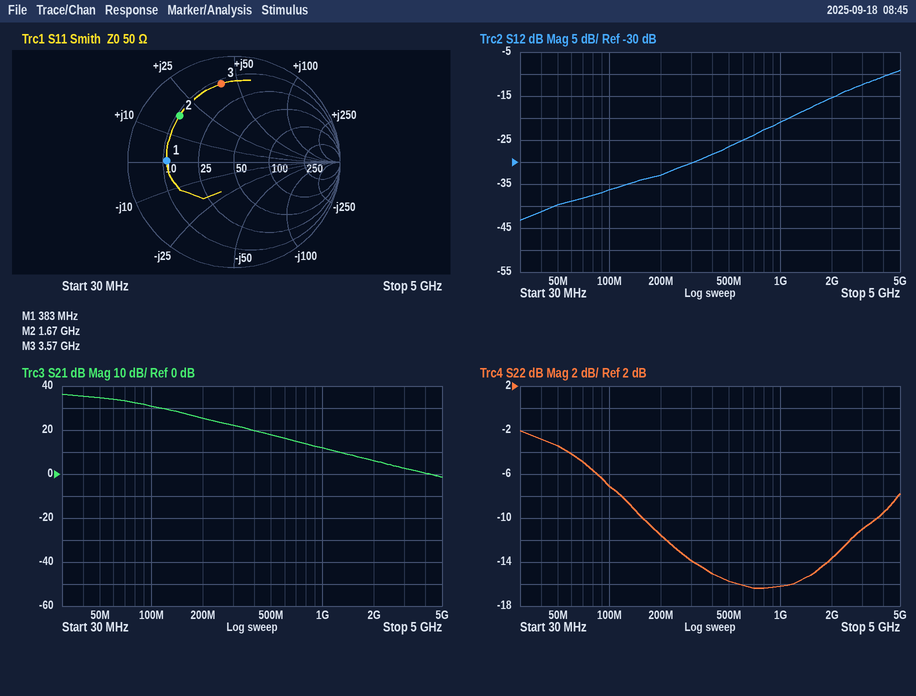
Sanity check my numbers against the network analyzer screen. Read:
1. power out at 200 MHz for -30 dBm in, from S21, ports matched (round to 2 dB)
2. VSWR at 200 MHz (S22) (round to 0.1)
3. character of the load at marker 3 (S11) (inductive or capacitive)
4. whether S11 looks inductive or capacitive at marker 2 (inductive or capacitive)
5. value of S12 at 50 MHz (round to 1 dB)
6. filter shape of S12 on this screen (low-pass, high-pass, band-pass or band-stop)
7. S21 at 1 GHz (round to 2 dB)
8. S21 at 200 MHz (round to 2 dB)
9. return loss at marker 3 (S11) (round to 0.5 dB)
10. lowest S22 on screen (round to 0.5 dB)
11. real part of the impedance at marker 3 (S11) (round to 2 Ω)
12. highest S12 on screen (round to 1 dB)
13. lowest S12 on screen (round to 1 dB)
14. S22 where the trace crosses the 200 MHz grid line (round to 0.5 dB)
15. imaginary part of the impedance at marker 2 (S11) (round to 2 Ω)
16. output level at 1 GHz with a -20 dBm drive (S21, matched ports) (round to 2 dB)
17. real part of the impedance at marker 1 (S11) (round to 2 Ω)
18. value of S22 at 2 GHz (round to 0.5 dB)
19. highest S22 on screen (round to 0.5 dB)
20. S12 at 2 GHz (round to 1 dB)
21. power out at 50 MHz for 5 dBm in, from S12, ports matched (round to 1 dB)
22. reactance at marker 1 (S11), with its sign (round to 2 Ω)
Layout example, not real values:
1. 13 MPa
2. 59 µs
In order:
1. -4 dBm
2. 1.7
3. inductive
4. inductive
5. -40 dB
6. high-pass
7. 12 dB
8. 26 dB
9. 2.5 dB
10. -16.5 dB
11. 12 Ω
12. -9 dB
13. -43 dB
14. -11.5 dB
15. +18 Ω
16. -8 dBm
17. 12 Ω
18. -13.5 dB
19. -2.0 dB
20. -15 dB
21. -35 dBm
22. 0 Ω
